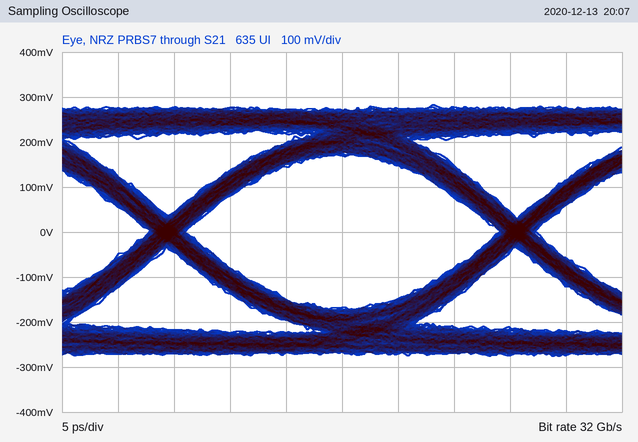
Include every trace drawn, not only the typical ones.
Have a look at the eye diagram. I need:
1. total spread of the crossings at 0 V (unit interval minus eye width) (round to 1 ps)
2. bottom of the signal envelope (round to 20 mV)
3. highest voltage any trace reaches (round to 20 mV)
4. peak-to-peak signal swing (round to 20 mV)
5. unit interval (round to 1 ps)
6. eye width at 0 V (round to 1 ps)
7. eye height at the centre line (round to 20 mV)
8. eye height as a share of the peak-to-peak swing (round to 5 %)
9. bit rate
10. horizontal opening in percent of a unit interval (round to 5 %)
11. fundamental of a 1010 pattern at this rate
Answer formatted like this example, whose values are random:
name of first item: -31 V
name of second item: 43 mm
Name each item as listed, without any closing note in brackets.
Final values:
total spread of the crossings at 0 V (unit interval minus eye width): 3 ps
bottom of the signal envelope: -280 mV
highest voltage any trace reaches: 280 mV
peak-to-peak signal swing: 560 mV
unit interval: 31 ps
eye width at 0 V: 28 ps
eye height at the centre line: 340 mV
eye height as a share of the peak-to-peak swing: 60 %
bit rate: 32 Gb/s
horizontal opening in percent of a unit interval: 90 %
fundamental of a 1010 pattern at this rate: 16 GHz
